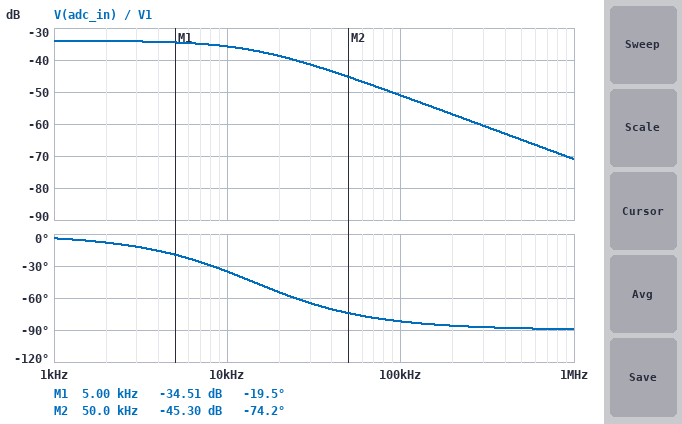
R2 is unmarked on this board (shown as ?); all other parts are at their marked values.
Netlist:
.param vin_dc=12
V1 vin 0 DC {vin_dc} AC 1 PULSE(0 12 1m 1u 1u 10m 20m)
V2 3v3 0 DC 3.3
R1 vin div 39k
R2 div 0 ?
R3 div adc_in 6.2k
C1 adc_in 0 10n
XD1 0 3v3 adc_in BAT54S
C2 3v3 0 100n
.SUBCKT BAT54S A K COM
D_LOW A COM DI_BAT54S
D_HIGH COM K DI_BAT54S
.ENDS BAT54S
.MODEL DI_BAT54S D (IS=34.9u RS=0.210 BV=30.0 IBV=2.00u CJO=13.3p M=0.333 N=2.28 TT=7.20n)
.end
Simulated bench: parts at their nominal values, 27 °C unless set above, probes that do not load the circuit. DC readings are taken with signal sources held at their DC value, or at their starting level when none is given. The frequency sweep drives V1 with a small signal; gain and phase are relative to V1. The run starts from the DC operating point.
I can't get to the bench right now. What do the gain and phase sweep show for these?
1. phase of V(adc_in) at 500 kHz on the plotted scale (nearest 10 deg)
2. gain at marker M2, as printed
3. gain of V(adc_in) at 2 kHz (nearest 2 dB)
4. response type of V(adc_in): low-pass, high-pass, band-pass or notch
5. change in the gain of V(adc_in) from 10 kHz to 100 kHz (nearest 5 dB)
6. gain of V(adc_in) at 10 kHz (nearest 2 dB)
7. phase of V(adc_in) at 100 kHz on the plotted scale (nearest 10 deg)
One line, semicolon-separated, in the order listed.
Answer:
-90 deg; -45.30 dB; -34 dB; low-pass; -15 dB; -36 dB; -80 deg
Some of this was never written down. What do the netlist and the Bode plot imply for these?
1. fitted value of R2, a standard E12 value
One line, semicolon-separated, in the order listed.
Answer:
22 kΩ
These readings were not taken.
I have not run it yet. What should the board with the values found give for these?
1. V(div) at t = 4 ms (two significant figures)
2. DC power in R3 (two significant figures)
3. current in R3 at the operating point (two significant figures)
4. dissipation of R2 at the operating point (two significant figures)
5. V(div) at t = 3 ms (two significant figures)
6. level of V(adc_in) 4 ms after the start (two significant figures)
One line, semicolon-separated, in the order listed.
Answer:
3.6 V; 15 µW; 50 µA; 600 µW; 3.6 V; 3.3 V
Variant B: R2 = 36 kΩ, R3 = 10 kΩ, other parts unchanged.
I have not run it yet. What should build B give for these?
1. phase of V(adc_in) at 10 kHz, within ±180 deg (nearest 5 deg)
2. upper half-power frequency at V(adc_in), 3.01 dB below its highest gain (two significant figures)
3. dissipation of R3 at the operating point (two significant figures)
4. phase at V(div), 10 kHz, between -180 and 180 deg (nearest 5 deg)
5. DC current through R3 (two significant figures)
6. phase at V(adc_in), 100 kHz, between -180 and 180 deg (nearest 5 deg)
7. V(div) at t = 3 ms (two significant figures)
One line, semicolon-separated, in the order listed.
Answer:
-25 deg; 23 kHz; 70 µW; 0 deg; 84 µA; -75 deg; 4.2 V
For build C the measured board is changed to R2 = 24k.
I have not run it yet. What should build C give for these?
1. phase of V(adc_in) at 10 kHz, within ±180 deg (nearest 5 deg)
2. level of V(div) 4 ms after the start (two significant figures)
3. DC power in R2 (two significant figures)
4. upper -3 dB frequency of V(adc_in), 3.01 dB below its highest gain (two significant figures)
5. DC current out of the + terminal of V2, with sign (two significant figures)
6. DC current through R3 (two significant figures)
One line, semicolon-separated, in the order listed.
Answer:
-30 deg; 3.7 V; 570 µW; 17 kHz; -24 µA; 59 µA
